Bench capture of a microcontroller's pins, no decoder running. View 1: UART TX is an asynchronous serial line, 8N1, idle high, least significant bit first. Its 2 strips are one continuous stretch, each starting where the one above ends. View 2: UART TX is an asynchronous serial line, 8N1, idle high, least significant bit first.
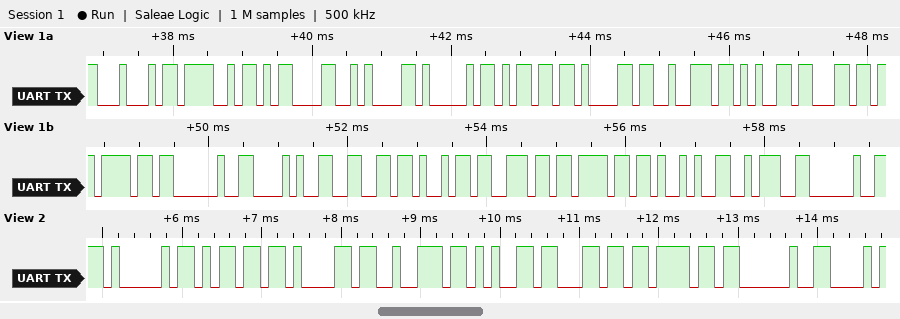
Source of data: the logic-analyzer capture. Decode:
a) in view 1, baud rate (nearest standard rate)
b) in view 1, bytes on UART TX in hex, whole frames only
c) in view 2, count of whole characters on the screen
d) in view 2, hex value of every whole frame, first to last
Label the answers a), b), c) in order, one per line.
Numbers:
a) 9600 baud
b) 0x44 0x4F 0x0D 0x0A 0x41 0x6D 0x61 0x72 0x65 0x6C 0x6F 0x20 0x28 0x66 0x69 0x6E 0x6F 0x29 0x3A 0x20
c) 8
d) 41 6D 61 72 65 6C 6F 20
